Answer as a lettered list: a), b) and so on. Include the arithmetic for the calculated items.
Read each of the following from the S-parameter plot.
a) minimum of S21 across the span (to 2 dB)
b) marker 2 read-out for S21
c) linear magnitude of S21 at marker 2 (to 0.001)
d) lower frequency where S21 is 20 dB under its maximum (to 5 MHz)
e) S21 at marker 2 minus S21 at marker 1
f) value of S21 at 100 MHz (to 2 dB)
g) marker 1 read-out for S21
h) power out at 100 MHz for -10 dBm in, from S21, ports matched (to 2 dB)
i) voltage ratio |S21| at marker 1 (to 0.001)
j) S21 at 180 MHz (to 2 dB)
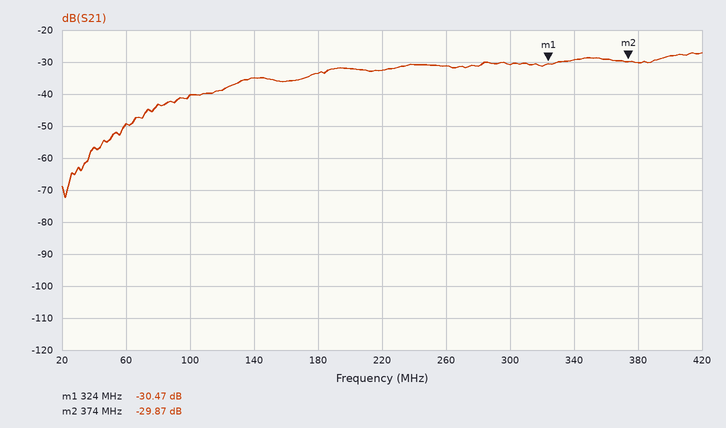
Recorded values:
a) -72 dB
b) -29.87 dB
c) 10^(-29.87/20) ≈ 0.032
d) 70 MHz
e) -29.87 − (-30.47) = 0.60 dB
f) -40 dB
g) -30.47 dB
h) -10 dBm + (-40 dB) = -50 dBm
i) 10^(-30.47/20) ≈ 0.030
j) -34 dB
